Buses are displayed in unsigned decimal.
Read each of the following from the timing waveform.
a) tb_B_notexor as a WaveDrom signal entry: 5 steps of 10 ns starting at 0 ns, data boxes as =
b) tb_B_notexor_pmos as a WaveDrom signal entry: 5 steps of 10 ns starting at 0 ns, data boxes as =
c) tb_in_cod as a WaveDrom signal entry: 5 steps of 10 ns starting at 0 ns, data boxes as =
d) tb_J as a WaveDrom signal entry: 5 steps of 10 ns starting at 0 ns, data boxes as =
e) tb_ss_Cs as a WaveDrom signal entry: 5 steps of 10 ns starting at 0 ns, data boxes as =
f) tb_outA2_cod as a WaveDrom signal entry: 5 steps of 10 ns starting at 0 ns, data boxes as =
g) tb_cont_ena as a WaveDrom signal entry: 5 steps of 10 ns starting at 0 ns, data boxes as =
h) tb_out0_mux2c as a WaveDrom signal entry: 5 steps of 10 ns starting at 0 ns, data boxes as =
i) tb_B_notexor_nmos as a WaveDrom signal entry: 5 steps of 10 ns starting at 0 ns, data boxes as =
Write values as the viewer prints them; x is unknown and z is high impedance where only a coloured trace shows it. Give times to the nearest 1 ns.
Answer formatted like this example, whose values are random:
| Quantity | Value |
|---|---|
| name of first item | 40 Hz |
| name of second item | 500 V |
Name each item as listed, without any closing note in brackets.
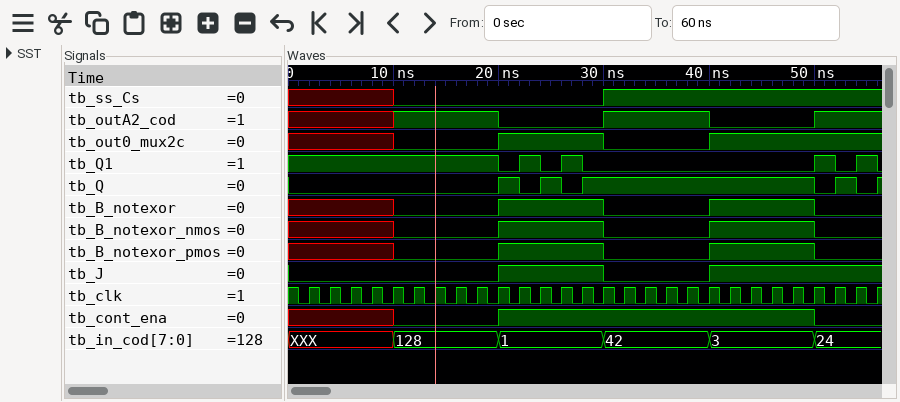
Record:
| Quantity | Value |
|---|---|
| tb_B_notexor as a WaveDrom signal entry: 5 steps of 10 ns starting at 0 ns, data boxes as = | {name: 'tb_B_notexor', wave: 'x0101'} |
| tb_B_notexor_pmos as a WaveDrom signal entry: 5 steps of 10 ns starting at 0 ns, data boxes as = | {name: 'tb_B_notexor_pmos', wave: 'x0101'} |
| tb_in_cod as a WaveDrom signal entry: 5 steps of 10 ns starting at 0 ns, data boxes as = | {name: 'tb_in_cod', wave: 'x====', data: '128 1 42 3'} |
| tb_J as a WaveDrom signal entry: 5 steps of 10 ns starting at 0 ns, data boxes as = | {name: 'tb_J', wave: '0.101'} |
| tb_ss_Cs as a WaveDrom signal entry: 5 steps of 10 ns starting at 0 ns, data boxes as = | {name: 'tb_ss_Cs', wave: 'x0.1.'} |
| tb_outA2_cod as a WaveDrom signal entry: 5 steps of 10 ns starting at 0 ns, data boxes as = | {name: 'tb_outA2_cod', wave: 'x1010'} |
| tb_cont_ena as a WaveDrom signal entry: 5 steps of 10 ns starting at 0 ns, data boxes as = | {name: 'tb_cont_ena', wave: 'x01..'} |
| tb_out0_mux2c as a WaveDrom signal entry: 5 steps of 10 ns starting at 0 ns, data boxes as = | {name: 'tb_out0_mux2c', wave: 'x0101'} |
| tb_B_notexor_nmos as a WaveDrom signal entry: 5 steps of 10 ns starting at 0 ns, data boxes as = | {name: 'tb_B_notexor_nmos', wave: 'x0101'} |
